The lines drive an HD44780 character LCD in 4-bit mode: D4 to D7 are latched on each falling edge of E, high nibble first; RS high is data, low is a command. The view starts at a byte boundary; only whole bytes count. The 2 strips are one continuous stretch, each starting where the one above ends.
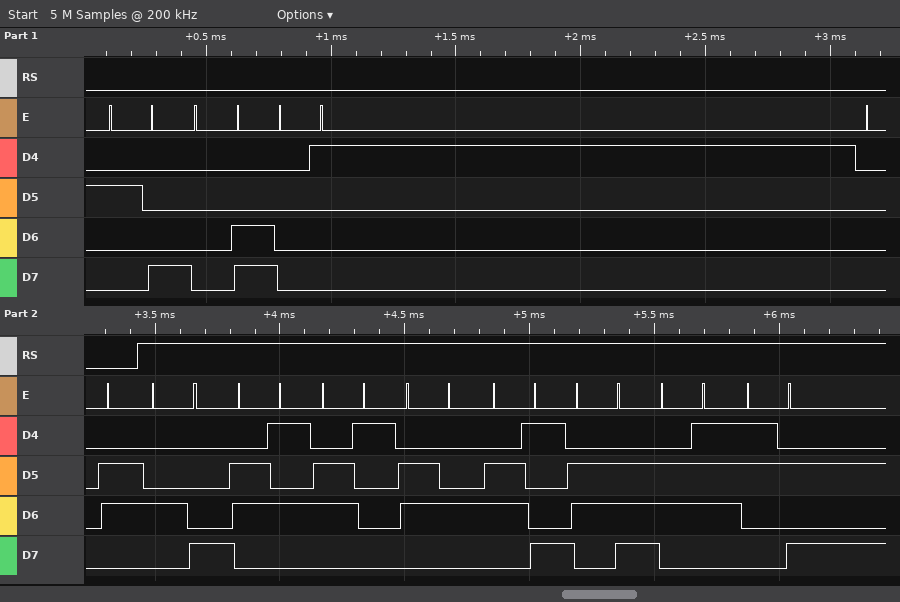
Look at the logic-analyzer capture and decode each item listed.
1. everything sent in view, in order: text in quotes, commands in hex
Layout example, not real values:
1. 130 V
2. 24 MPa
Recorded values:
1. 0x28 0x0C 0x01 0x06 "Heading:"
